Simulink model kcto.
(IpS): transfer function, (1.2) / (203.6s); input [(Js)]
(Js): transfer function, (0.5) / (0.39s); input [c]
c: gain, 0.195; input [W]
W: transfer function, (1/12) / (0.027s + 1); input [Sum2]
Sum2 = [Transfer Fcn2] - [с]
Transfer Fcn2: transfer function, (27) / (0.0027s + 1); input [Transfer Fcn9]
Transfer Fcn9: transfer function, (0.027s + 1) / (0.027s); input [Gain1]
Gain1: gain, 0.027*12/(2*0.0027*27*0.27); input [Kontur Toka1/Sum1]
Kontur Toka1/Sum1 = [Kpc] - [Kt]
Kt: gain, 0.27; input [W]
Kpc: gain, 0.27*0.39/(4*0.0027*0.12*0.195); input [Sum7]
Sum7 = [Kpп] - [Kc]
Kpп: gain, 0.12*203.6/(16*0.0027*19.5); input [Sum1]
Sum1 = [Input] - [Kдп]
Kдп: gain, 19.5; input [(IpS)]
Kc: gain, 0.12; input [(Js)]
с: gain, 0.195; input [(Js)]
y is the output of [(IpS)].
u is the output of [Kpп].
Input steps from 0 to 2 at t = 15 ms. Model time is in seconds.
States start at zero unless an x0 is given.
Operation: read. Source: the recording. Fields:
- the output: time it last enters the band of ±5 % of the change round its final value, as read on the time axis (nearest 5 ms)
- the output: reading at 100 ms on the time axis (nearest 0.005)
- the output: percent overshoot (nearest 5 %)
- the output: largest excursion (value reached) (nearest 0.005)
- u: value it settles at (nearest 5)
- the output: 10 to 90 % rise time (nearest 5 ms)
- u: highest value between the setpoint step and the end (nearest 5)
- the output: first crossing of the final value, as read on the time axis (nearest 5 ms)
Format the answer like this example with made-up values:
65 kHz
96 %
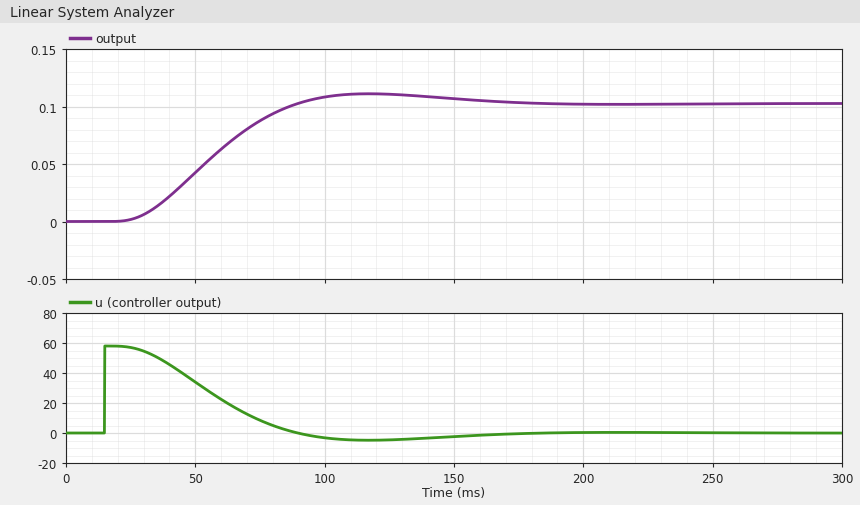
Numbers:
145 ms
0.110
10 %
0.110
0
45 ms
60
90 ms
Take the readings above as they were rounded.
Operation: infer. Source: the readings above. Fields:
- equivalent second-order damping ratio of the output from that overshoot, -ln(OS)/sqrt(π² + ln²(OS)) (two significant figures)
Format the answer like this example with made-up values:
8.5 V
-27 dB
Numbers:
0.59
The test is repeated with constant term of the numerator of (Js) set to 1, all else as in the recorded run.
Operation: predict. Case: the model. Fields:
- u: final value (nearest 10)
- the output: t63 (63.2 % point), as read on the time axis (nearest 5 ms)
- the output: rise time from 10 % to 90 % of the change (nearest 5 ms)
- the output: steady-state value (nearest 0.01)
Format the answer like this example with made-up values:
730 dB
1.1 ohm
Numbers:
0
50 ms
50 ms
0.10
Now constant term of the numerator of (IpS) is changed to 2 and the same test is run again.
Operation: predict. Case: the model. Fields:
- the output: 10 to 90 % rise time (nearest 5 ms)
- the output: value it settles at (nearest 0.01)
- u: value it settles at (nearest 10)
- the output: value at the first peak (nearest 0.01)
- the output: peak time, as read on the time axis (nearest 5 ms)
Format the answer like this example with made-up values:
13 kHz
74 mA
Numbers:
30 ms
0.10
0
0.13
85 ms
